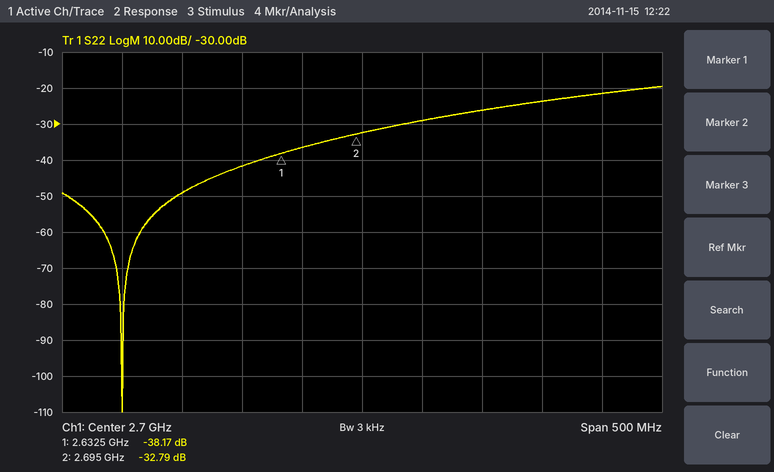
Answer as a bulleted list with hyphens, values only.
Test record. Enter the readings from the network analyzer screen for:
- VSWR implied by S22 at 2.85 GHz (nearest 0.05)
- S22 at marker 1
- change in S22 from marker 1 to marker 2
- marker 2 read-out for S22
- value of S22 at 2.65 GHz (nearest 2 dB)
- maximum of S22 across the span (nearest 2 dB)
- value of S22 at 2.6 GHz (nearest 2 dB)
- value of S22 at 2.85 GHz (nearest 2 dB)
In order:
- 1.15
- -38.17 dB
- 5.38 dB
- -32.79 dB
- -36 dB
- -20 dB
- -42 dB
- -24 dB
